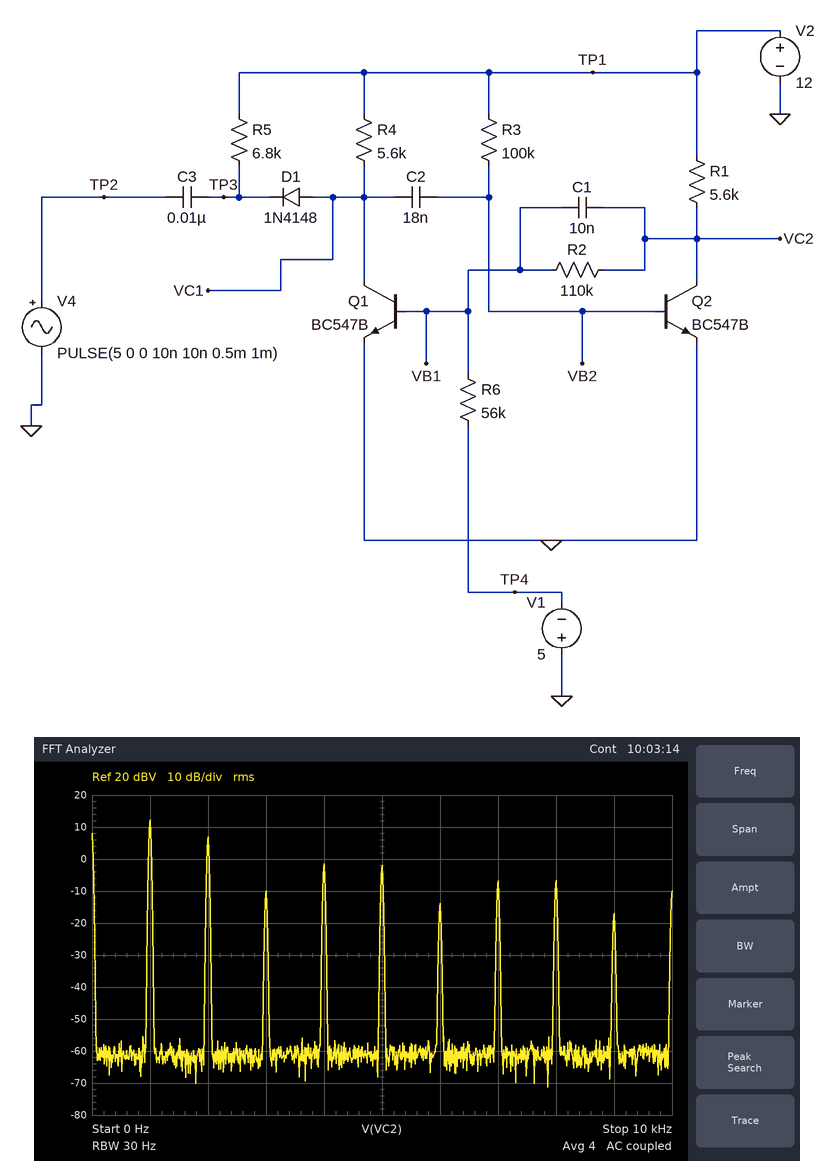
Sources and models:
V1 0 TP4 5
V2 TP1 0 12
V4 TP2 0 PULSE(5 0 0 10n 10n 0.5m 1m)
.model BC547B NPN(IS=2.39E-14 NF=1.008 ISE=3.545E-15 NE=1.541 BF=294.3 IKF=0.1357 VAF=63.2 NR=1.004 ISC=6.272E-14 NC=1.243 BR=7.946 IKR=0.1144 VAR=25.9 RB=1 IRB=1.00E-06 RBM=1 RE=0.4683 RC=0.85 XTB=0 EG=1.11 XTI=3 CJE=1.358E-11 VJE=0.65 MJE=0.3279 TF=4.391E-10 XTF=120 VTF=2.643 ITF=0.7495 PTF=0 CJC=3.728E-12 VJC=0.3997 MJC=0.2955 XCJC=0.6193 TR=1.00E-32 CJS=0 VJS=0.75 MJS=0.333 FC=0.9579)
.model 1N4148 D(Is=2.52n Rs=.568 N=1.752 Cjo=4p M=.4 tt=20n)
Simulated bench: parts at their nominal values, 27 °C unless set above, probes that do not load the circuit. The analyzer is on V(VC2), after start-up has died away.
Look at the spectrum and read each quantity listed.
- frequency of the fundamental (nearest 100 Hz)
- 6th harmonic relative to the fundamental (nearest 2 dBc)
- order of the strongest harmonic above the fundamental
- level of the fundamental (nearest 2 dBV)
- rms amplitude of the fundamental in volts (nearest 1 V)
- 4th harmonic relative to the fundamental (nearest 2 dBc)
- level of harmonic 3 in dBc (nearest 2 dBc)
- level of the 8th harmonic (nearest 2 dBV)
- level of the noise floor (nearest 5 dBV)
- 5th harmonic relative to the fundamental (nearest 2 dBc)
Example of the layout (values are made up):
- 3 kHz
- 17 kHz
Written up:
- 1.0 kHz
- -26 dBc
- 2
- 12 dBV
- 4 V
- -14 dBc
- -22 dBc
- -6 dBV
- -60 dBV
- -14 dBc
